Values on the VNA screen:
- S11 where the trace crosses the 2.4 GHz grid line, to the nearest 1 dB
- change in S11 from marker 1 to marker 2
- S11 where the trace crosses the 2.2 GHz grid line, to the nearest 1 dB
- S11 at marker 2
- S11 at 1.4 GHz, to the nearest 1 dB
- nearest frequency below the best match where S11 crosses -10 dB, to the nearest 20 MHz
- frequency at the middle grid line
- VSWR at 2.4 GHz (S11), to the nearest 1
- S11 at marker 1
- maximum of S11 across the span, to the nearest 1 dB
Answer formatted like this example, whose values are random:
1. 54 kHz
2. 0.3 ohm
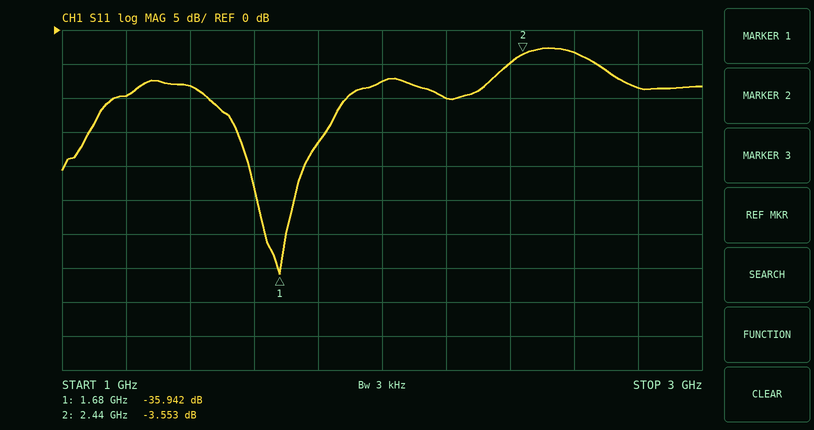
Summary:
1. -5 dB
2. 32.389 dB
3. -10 dB
4. -3.553 dB
5. -8 dB
6. 1.46 GHz
7. 2 GHz
8. 4
9. -35.942 dB
10. -3 dB
